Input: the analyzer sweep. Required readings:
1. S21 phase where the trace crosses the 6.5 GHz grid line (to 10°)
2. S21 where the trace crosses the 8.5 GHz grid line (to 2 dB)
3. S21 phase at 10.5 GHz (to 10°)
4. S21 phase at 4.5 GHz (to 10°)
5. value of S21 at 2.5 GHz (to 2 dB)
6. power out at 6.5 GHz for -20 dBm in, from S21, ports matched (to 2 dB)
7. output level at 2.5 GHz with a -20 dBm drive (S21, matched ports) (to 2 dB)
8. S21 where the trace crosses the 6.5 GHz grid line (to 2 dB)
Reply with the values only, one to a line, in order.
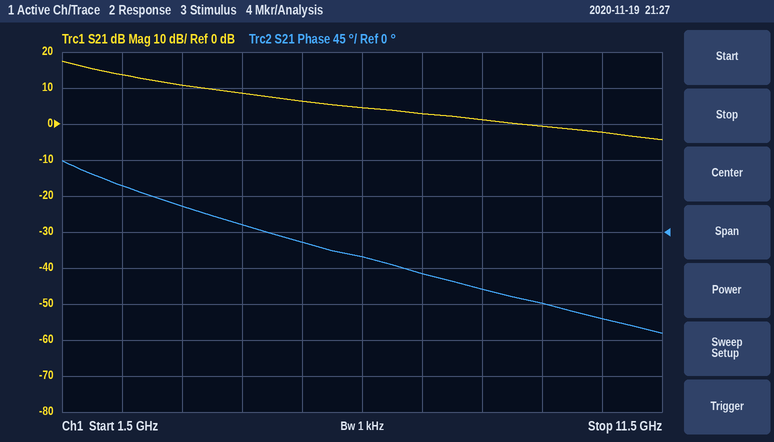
-30°
2 dB
-110°
10°
14 dB
-16 dBm
-6 dBm
4 dB
